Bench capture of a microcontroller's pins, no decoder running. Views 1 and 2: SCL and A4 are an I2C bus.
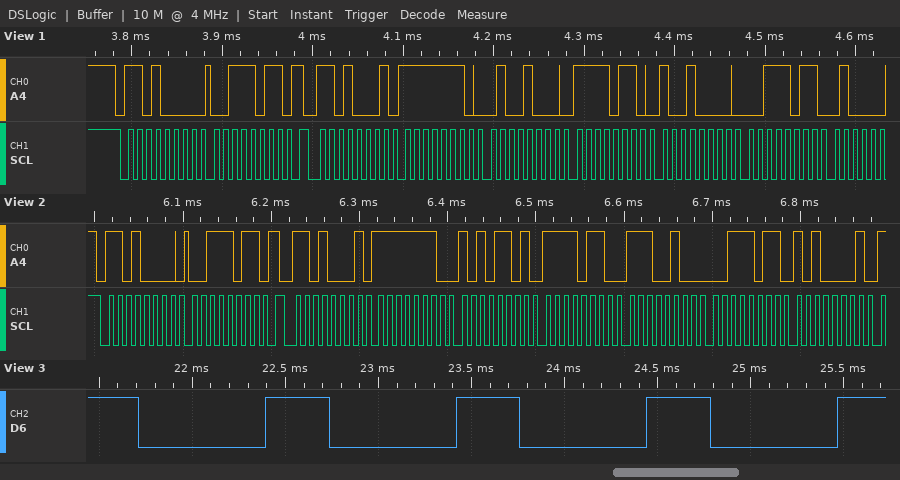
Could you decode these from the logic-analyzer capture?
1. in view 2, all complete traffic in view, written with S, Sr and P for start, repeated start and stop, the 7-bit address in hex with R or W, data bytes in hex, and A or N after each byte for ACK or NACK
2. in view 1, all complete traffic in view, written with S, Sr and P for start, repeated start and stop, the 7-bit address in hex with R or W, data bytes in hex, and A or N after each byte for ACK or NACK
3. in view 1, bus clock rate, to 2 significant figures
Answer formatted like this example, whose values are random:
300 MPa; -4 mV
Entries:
S 68W A 3B A Sr 68R A FE A AD A F6 A E4 A 3B A A1 A; S 68W A 3B A Sr 68R A FE A 48 A F6 A 90 A 3B A; 100 kHz
